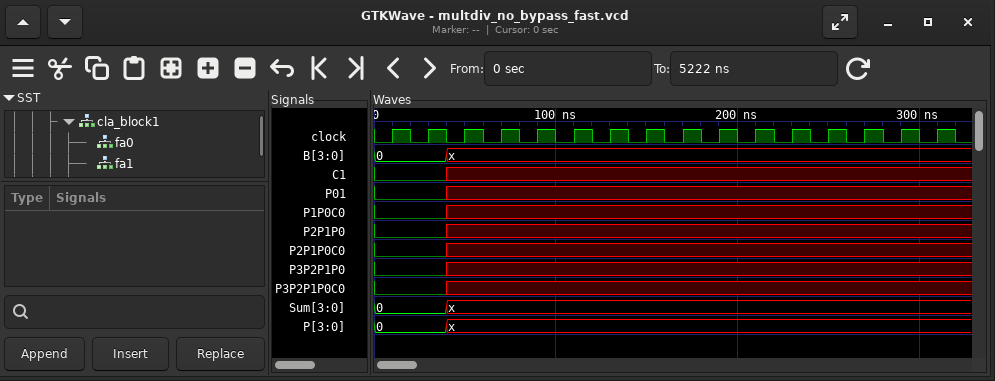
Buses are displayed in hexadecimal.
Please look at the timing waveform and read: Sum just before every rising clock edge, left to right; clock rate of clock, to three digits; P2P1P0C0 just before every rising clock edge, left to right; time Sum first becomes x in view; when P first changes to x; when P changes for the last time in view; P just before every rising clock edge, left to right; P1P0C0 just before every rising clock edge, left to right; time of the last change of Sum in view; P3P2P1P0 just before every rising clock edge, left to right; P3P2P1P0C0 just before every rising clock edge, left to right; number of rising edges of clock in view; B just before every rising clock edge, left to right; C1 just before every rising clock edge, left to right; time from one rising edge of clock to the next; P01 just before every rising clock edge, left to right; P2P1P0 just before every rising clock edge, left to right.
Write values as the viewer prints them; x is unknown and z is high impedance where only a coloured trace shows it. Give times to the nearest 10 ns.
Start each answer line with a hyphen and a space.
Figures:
- 0, 0, x, x, x, x, x, x, x, x, x, x, x, x, x, x
- 50.0 MHz
- 0 0 x x x x x x x x x x x x x x
- 40 ns
- 40 ns
- 40 ns
- 0, 0, x, x, x, x, x, x, x, x, x, x, x, x, x, x
- 0 0 x x x x x x x x x x x x x x
- 40 ns
- 0 0 x x x x x x x x x x x x x x
- 0 0 x x x x x x x x x x x x x x
- 16
- 0, 0, x, x, x, x, x, x, x, x, x, x, x, x, x, x
- 0 0 x x x x x x x x x x x x x x
- 20 ns
- 0 0 x x x x x x x x x x x x x x
- 0 0 x x x x x x x x x x x x x x
